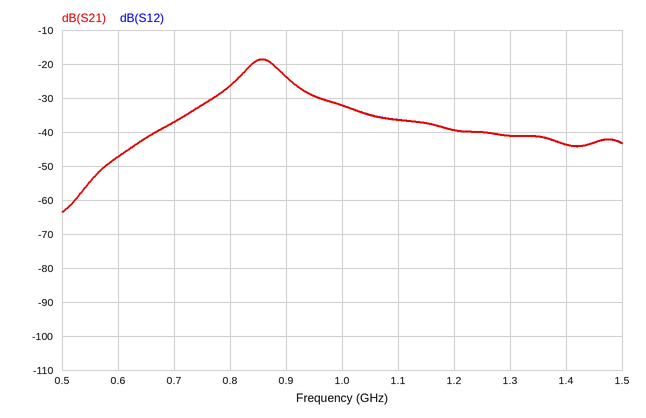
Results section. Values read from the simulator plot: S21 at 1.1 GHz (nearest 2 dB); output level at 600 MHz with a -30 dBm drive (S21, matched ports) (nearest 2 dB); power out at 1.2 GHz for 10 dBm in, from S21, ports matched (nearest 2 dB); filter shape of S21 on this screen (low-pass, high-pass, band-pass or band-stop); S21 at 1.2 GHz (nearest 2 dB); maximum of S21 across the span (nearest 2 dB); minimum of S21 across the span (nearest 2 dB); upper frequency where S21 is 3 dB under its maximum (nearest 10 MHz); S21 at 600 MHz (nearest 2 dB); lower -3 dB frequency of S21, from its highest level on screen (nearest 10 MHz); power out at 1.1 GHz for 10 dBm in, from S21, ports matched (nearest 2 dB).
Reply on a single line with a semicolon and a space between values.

-36 dB; -78 dBm; -30 dBm; band-pass; -40 dB; -18 dB; -64 dB; 890 MHz; -48 dB; 830 MHz; -26 dBm
